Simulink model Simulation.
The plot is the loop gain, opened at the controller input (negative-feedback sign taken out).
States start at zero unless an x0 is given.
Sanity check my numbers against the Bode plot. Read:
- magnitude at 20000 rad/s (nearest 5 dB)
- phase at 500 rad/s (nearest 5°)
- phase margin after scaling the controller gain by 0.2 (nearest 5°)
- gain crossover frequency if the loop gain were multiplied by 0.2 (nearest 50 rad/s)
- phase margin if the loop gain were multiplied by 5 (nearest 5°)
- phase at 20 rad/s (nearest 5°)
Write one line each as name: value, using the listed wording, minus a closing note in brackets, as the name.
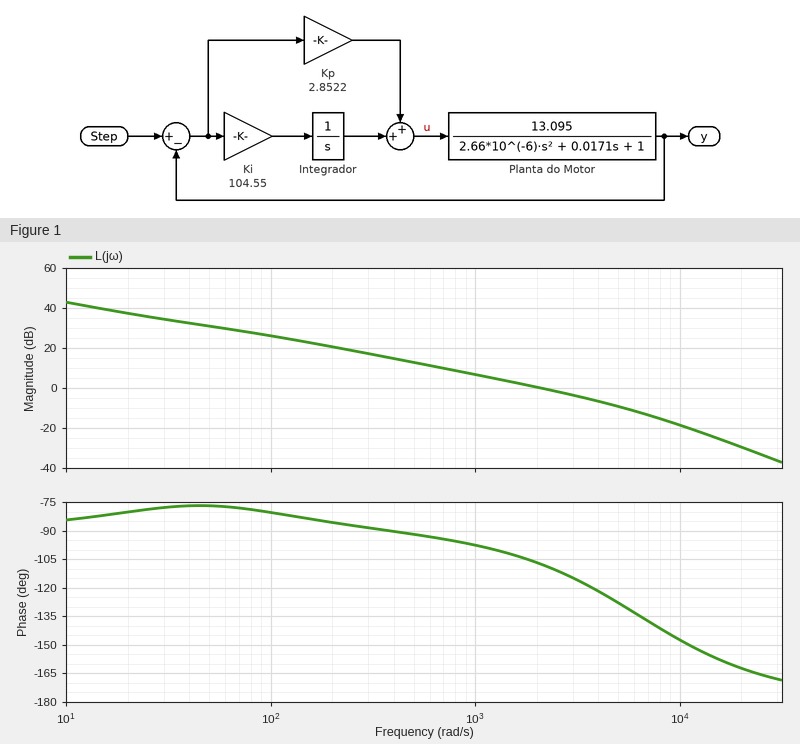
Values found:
magnitude at 20000 rad/s: -30 dB
phase at 500 rad/s: -90°
phase margin after scaling the controller gain by 0.2: 90°
gain crossover frequency if the loop gain were multiplied by 0.2: 450 rad/s
phase margin if the loop gain were multiplied by 5: 40°
phase at 20 rad/s: -80°
